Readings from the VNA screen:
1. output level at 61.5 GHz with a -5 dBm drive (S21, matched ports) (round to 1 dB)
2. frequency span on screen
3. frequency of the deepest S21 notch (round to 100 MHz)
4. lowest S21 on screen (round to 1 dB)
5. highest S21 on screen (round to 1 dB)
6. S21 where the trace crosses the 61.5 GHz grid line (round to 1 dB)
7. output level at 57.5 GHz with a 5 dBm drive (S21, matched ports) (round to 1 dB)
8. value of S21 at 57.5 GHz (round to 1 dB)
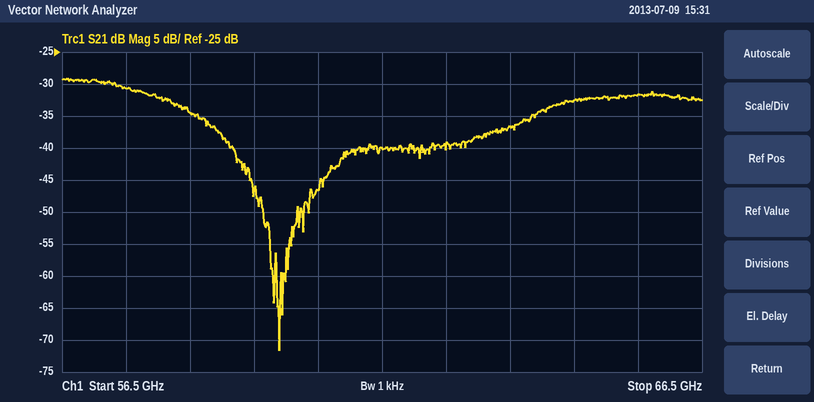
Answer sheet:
-45 dBm
10 GHz
59.9 GHz
-72 dB
-29 dB
-40 dB
-26 dBm
-31 dB
